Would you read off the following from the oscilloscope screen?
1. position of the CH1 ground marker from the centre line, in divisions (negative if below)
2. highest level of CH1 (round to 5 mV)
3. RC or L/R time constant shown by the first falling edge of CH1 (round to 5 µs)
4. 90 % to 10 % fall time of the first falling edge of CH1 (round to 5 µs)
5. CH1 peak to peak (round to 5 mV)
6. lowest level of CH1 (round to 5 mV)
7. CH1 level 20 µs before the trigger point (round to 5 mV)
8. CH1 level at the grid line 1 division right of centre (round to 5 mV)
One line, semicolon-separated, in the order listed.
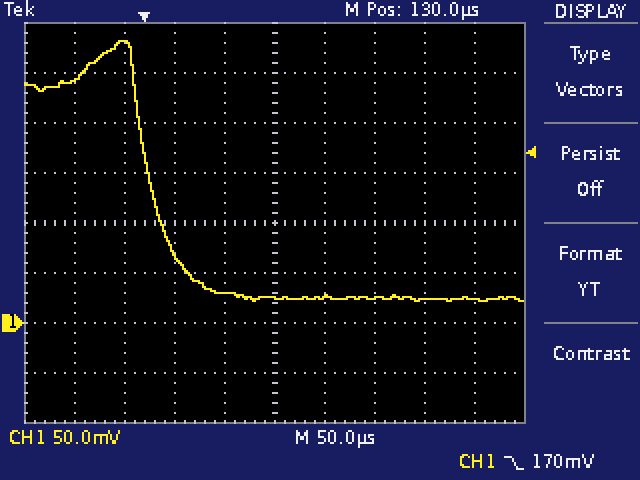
-2.0 div; 280 mV; 25 µs; 55 µs; 260 mV; 20 mV; 280 mV; 25 mV
